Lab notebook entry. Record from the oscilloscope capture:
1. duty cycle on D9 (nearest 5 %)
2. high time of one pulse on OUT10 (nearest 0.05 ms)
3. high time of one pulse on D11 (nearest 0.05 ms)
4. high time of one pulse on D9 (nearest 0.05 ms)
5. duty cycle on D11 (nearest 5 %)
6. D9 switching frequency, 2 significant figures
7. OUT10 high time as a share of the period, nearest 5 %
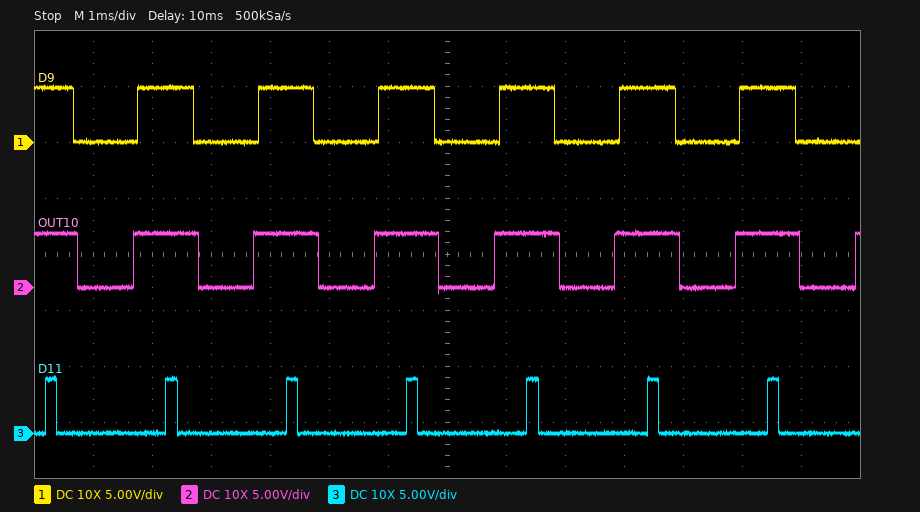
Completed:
45 %
1.10 ms
0.20 ms
0.95 ms
10 %
490 Hz
55 %
